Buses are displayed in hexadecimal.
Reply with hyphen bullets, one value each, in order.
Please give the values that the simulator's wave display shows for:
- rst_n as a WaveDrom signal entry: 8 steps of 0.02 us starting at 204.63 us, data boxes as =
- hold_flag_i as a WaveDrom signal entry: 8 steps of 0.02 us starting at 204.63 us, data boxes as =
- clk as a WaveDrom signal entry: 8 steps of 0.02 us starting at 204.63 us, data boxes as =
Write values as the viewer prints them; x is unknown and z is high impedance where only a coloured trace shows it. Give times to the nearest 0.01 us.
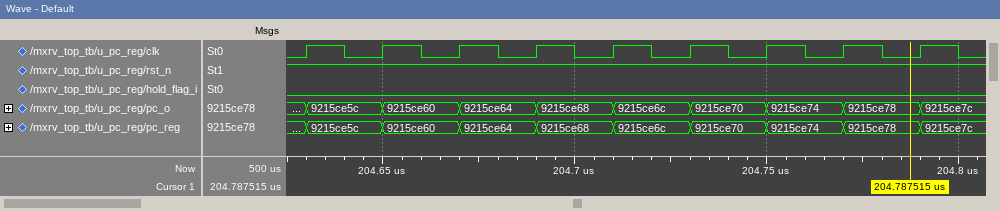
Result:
- {name: 'rst_n', wave: '1.......'}
- {name: 'hold_flag_i', wave: '0.......'}
- {name: 'clk', wave: 'p.......'}
